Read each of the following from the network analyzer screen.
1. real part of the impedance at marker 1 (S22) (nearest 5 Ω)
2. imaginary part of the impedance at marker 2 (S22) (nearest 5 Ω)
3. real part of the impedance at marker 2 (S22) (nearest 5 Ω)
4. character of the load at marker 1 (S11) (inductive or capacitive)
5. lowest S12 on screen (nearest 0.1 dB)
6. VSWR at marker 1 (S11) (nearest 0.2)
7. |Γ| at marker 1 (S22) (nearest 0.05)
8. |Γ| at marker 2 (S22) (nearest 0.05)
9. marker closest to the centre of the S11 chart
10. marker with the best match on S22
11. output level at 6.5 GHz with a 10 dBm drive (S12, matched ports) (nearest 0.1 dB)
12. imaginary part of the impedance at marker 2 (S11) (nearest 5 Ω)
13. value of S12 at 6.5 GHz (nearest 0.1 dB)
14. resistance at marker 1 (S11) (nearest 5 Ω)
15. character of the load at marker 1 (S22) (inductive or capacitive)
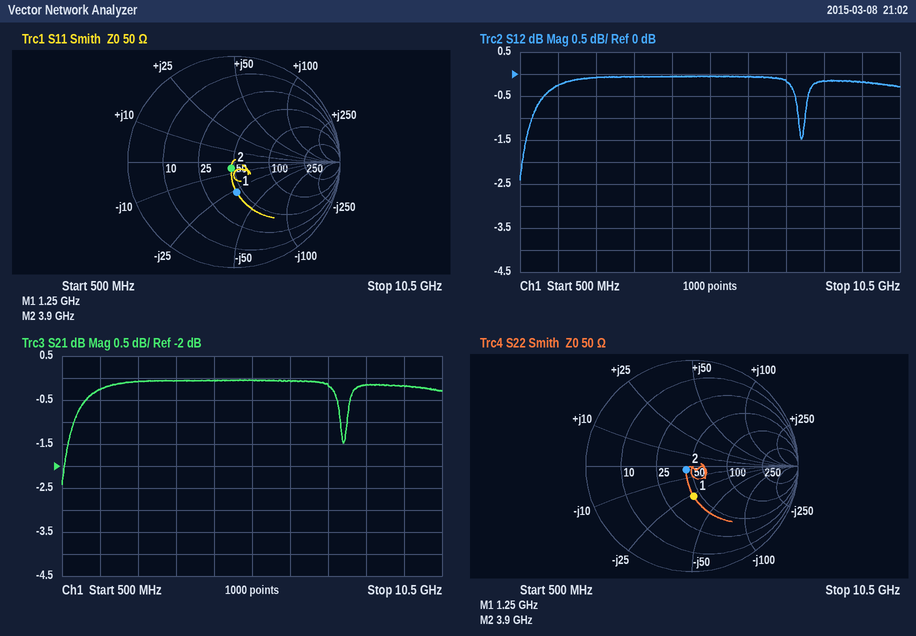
45 Ω
-5 Ω
45 Ω
capacitive
-2.4 dB
1.8
0.30
0.05
marker 2
marker 2
9.9 dBm
-5 Ω
-0.1 dB
45 Ω
capacitive
